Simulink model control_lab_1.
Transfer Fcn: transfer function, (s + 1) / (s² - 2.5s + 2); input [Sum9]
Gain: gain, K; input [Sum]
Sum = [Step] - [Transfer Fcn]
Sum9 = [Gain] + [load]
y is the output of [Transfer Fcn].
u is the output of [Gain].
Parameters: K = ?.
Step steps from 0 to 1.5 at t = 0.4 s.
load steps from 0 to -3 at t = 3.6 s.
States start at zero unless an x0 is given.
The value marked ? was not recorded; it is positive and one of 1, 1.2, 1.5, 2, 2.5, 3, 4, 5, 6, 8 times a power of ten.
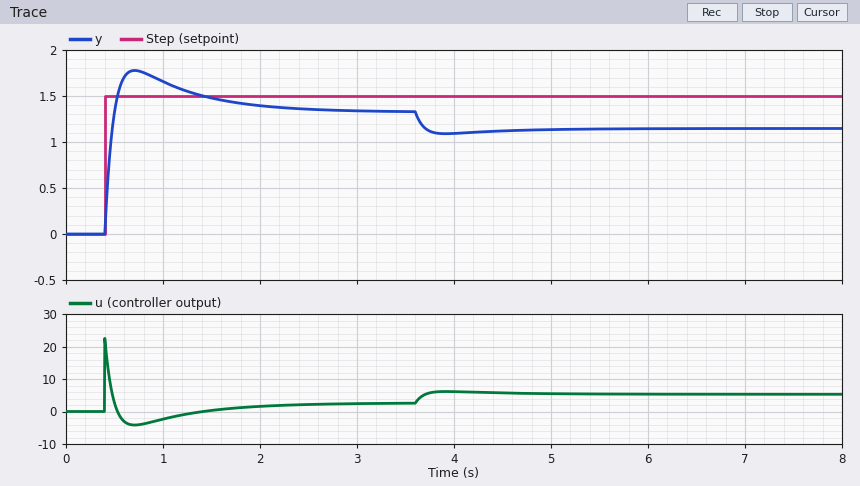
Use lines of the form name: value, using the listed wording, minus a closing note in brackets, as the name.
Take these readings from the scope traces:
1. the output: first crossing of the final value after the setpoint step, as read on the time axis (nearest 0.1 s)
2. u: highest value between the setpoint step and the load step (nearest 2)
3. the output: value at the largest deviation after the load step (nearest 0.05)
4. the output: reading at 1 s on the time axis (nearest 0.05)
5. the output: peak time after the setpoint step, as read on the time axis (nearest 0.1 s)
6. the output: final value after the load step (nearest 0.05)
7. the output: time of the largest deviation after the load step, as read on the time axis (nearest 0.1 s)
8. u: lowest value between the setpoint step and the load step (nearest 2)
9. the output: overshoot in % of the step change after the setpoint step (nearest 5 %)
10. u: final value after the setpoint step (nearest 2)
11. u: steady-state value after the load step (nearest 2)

the output: first crossing of the final value after the setpoint step, as read on the time axis: 0.5 s
u: highest value between the setpoint step and the load step: 22
the output: value at the largest deviation after the load step: 1.10
the output: reading at 1 s on the time axis: 1.65
the output: peak time after the setpoint step, as read on the time axis: 0.7 s
the output: final value after the load step: 1.15
the output: time of the largest deviation after the load step, as read on the time axis: 3.9 s
u: lowest value between the setpoint step and the load step: -4
the output: overshoot in % of the step change after the setpoint step: 35 %
u: final value after the setpoint step: 2
u: steady-state value after the load step: 6
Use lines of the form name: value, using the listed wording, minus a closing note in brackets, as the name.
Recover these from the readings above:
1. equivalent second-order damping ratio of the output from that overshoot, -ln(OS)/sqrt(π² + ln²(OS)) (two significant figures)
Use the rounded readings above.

equivalent second-order damping ratio of the output from that overshoot, -ln(OS)/sqrt(π² + ln²(OS)): 0.32
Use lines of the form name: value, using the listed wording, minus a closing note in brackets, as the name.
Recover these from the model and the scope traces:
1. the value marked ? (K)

the value marked ?: 15
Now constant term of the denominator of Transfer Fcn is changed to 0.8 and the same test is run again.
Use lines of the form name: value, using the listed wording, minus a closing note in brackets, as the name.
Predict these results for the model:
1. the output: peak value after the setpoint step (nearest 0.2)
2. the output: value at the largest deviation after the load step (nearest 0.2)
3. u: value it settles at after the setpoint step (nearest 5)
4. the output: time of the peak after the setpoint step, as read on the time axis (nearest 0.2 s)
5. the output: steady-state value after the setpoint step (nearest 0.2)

the output: peak value after the setpoint step: 1.8
the output: value at the largest deviation after the load step: 1.2
u: value it settles at after the setpoint step: 0
the output: time of the peak after the setpoint step, as read on the time axis: 0.8 s
the output: steady-state value after the setpoint step: 1.4
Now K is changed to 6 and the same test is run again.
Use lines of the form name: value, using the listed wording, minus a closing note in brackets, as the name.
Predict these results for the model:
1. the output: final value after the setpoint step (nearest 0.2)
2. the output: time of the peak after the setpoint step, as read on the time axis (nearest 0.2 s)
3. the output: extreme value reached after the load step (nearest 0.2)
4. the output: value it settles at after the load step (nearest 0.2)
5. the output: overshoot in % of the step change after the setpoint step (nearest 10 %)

the output: final value after the setpoint step: 1.2
the output: time of the peak after the setpoint step, as read on the time axis: 1.0 s
the output: extreme value reached after the load step: 0.4
the output: value it settles at after the load step: 0.8
the output: overshoot in % of the step change after the setpoint step: 90 %
